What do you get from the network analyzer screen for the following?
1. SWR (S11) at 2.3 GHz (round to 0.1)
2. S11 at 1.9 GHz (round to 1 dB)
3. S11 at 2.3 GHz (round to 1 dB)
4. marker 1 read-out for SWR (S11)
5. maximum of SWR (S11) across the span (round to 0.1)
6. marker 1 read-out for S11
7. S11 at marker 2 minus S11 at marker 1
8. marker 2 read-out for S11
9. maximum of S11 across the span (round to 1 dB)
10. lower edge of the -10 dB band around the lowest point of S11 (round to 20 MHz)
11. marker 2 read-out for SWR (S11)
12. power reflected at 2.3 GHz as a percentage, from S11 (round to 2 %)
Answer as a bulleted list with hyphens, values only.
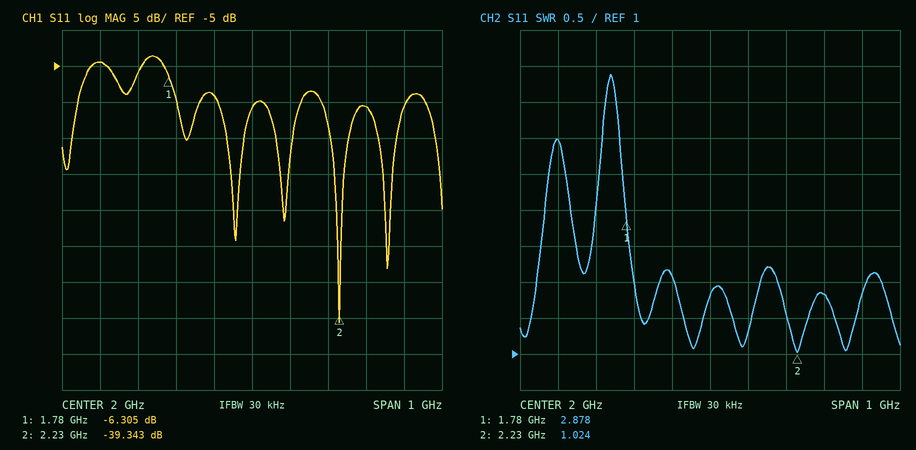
- 1.8
- -9 dB
- -11 dB
- 2.878
- 4.9
- -6.305 dB
- -33.038 dB
- -39.343 dB
- -4 dB
- 2.18 GHz
- 1.024
- 8 %
